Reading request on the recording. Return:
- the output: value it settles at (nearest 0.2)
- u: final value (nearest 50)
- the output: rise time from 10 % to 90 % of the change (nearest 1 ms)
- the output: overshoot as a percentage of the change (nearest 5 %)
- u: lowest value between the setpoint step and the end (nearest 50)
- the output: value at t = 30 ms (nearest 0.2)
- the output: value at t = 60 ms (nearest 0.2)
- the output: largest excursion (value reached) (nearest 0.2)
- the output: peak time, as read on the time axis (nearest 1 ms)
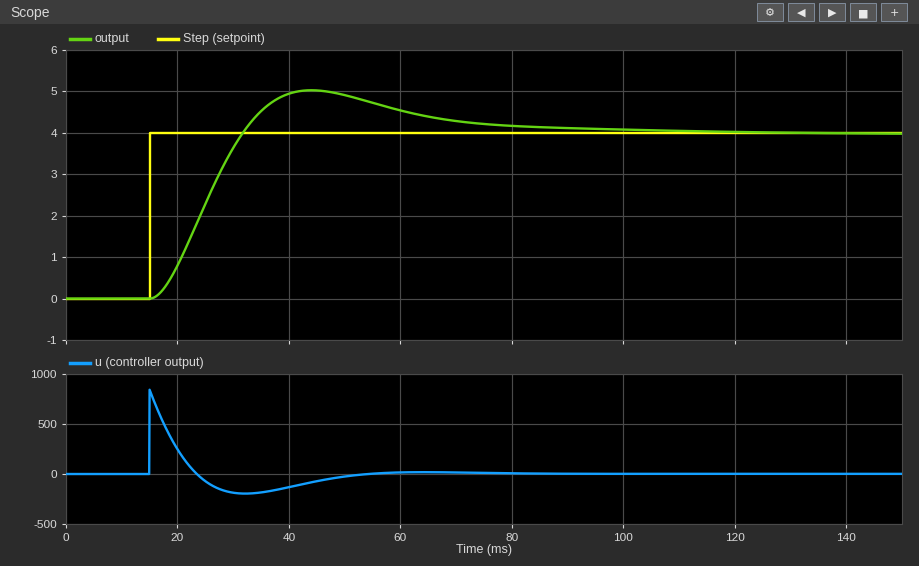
4.0
0
11 ms
25 %
-200
3.6
4.6
5.0
44 ms
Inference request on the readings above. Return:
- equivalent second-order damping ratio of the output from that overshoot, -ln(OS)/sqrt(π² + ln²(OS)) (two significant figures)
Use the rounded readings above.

0.40
